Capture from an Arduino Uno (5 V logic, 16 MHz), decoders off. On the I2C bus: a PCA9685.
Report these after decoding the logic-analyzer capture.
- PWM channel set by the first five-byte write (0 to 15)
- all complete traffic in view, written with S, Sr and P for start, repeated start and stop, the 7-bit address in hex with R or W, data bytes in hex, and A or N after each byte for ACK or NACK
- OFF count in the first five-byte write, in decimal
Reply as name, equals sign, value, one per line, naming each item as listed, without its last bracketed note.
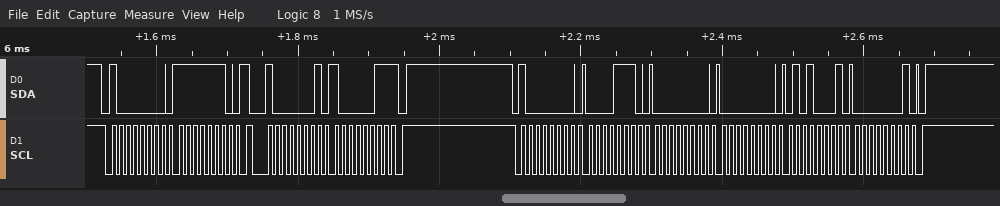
PWM channel set by the first five-byte write = 2
all complete traffic in view, written with S, Sr and P for start, repeated start and stop, the 7-bit address in hex with R or W, data bytes in hex, and A or N after each byte for ACK or NACK = S 40W A FE A Sr 40R A 83 N P S 40W A 0E A 00 A 00 A 51 A 01 A P
OFF count in the first five-byte write, in decimal = 337
